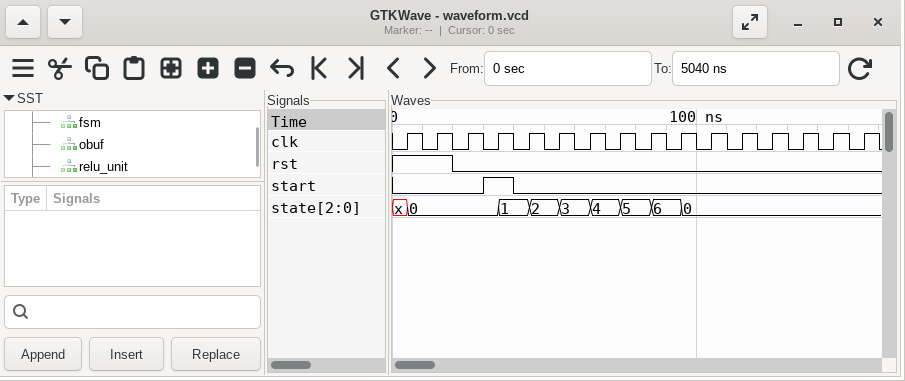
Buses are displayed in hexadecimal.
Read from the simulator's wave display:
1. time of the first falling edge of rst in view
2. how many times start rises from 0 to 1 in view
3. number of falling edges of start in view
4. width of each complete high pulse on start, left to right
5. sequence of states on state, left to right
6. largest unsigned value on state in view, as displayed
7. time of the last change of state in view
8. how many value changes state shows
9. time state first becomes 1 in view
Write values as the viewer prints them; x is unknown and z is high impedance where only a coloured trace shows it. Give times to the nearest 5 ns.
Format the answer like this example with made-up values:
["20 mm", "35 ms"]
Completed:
["20 ns", "1", "1", "10 ns", "x, 0, 1, 2, 3, 4, 5, 6, 0", "6", "95 ns", "8", "35 ns"]
